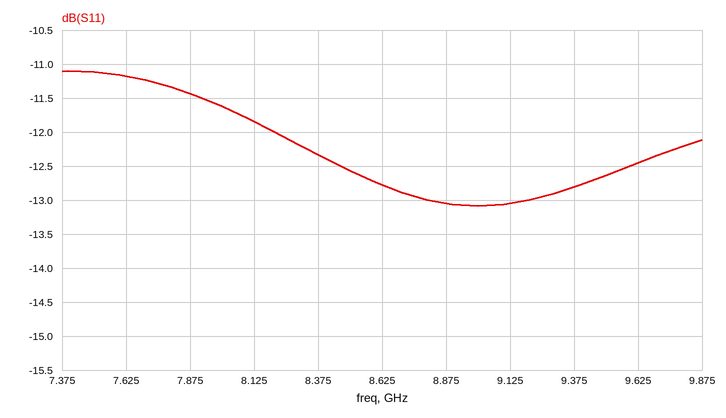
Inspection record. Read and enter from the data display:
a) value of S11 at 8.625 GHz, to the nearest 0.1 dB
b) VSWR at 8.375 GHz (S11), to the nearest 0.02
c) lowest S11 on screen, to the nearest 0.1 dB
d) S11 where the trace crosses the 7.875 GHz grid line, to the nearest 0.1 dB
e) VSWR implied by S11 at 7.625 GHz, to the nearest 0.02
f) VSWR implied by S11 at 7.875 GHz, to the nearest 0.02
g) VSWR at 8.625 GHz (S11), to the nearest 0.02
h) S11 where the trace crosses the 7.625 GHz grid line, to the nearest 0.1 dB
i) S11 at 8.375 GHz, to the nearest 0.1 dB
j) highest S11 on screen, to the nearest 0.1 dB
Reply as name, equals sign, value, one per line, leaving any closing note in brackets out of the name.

value of S11 at 8.625 GHz, to the nearest 0.1 dB = -12.8 dB
VSWR at 8.375 GHz (S11), to the nearest 0.02 = 1.64
lowest S11 on screen, to the nearest 0.1 dB = -13.1 dB
S11 where the trace crosses the 7.875 GHz grid line, to the nearest 0.1 dB = -11.4 dB
VSWR implied by S11 at 7.625 GHz, to the nearest 0.02 = 1.76
VSWR implied by S11 at 7.875 GHz, to the nearest 0.02 = 1.74
VSWR at 8.625 GHz (S11), to the nearest 0.02 = 1.60
S11 where the trace crosses the 7.625 GHz grid line, to the nearest 0.1 dB = -11.2 dB
S11 at 8.375 GHz, to the nearest 0.1 dB = -12.3 dB
highest S11 on screen, to the nearest 0.1 dB = -11.1 dB
